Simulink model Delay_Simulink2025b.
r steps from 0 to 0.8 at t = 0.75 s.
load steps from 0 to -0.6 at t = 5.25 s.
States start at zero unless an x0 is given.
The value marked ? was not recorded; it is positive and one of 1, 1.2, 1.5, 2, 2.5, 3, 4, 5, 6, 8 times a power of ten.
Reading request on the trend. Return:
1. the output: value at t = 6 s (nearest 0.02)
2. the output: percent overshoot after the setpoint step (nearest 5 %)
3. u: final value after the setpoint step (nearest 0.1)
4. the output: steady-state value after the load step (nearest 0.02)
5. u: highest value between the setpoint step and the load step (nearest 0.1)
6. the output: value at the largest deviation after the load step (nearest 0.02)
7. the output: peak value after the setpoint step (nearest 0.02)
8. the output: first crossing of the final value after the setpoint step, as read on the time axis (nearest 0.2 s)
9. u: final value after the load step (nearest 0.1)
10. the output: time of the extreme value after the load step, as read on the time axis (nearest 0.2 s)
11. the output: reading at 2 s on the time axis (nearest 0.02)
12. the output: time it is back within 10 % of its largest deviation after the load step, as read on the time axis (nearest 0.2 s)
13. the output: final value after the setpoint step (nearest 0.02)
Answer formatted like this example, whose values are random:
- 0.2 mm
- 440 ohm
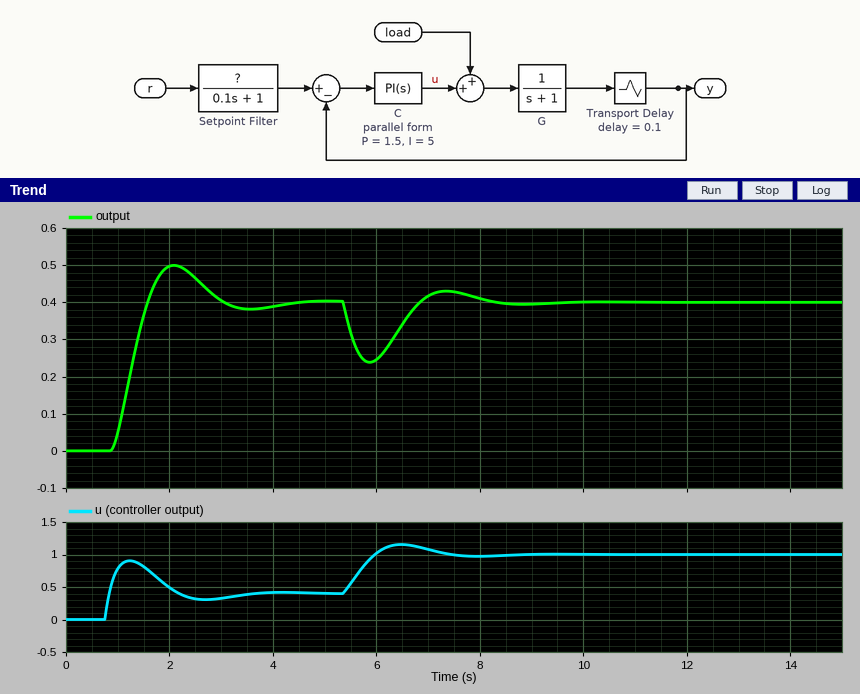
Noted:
- 0.24
- 25 %
- 0.4
- 0.40
- 0.9
- 0.24
- 0.50
- 1.6 s
- 1.0
- 5.8 s
- 0.50
- 7.8 s
- 0.40
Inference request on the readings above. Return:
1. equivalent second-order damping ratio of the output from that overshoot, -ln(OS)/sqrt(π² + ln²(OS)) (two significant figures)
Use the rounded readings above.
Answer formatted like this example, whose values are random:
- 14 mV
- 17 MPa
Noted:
- 0.40
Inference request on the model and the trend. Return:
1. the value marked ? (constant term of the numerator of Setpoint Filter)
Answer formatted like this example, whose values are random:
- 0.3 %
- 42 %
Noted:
- 0.5
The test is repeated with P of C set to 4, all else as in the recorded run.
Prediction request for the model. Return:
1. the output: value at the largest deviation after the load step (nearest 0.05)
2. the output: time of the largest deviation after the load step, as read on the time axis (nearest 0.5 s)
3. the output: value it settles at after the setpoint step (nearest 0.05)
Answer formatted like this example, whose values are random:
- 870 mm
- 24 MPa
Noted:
- 0.30
- 5.5 s
- 0.40
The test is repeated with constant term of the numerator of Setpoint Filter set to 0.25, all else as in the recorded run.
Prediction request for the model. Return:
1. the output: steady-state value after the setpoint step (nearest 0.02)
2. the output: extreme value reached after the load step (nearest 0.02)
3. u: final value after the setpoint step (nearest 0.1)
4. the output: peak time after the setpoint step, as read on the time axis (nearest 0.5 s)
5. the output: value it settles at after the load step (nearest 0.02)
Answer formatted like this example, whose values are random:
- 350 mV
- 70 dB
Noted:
- 0.20
- 0.04
- 0.2
- 2.0 s
- 0.20
